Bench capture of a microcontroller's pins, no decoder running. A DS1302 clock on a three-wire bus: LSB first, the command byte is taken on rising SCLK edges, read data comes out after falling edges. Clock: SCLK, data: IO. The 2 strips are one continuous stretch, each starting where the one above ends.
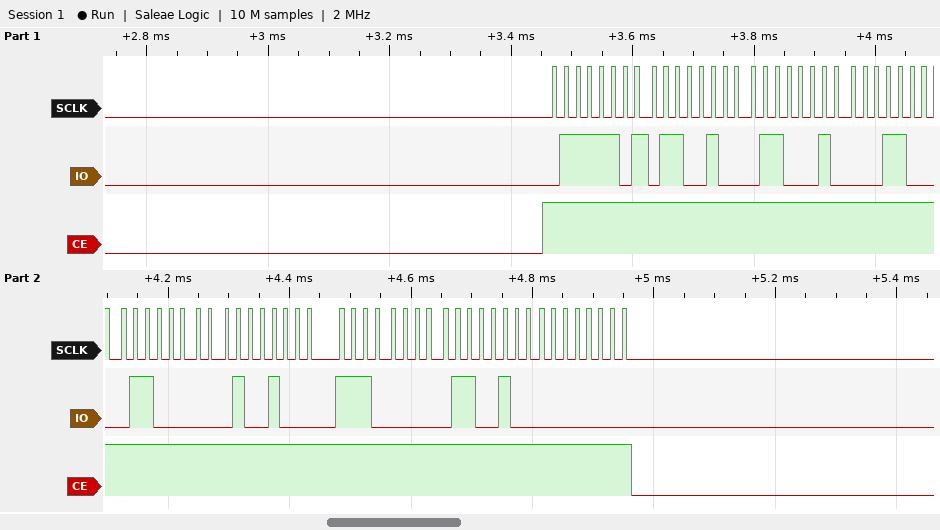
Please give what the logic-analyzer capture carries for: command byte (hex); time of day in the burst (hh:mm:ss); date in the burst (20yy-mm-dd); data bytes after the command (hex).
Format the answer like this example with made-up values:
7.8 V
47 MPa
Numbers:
0xBE
18:46:26
2026-12-06
26 46 18 06 12 07 26 00
